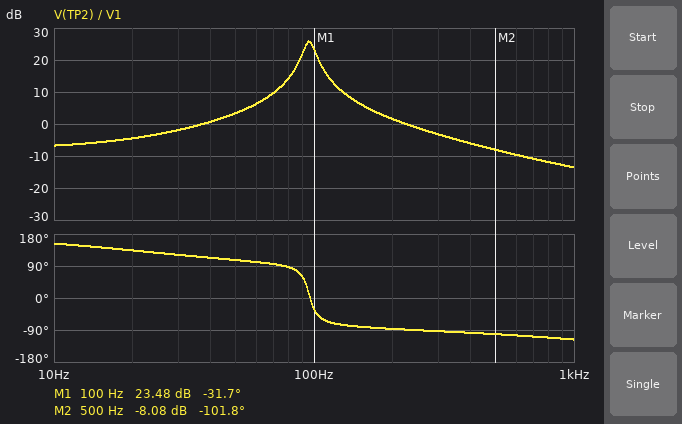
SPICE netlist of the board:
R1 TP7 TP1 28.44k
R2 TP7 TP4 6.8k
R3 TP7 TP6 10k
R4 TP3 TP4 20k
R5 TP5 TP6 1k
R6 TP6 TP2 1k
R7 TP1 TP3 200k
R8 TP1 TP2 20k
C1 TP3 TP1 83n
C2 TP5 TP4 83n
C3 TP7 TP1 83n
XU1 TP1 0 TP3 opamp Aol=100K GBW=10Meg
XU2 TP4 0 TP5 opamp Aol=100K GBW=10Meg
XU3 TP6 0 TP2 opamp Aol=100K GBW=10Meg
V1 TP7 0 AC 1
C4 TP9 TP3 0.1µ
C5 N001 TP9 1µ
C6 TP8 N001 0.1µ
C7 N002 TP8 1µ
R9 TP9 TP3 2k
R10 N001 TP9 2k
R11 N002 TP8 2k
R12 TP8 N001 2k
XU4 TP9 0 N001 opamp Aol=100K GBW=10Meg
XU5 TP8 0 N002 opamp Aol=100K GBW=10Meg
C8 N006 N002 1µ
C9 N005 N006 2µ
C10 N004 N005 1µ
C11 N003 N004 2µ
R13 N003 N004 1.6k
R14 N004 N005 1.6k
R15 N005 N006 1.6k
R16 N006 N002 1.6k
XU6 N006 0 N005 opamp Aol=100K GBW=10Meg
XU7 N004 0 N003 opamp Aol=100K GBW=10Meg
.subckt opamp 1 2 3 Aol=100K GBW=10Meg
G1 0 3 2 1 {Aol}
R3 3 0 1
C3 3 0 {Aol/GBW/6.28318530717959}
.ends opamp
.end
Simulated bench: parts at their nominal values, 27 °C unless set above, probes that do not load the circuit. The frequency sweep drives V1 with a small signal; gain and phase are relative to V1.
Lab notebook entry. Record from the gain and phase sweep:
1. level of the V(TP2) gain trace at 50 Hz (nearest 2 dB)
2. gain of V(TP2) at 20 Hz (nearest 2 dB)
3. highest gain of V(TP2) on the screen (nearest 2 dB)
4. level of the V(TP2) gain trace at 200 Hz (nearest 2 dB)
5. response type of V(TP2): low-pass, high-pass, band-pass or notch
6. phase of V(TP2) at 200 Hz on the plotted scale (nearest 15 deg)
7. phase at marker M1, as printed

4 dB
-4 dB
26 dB
2 dB
band-pass
-90 deg
-31.7 deg
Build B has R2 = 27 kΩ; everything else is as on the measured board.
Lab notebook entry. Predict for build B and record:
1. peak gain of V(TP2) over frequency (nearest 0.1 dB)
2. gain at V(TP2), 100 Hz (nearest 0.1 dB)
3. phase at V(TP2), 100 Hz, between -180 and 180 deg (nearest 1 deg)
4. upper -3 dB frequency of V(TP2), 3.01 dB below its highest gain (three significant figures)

15.5 dB
12.7 dB
78 deg
100 Hz
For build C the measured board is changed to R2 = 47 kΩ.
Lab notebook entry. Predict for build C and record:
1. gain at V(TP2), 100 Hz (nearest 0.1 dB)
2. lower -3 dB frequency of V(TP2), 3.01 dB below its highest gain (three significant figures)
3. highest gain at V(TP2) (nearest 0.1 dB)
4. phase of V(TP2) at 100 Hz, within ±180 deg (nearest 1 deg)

15.6 dB
90.9 Hz
18.2 dB
98 deg
